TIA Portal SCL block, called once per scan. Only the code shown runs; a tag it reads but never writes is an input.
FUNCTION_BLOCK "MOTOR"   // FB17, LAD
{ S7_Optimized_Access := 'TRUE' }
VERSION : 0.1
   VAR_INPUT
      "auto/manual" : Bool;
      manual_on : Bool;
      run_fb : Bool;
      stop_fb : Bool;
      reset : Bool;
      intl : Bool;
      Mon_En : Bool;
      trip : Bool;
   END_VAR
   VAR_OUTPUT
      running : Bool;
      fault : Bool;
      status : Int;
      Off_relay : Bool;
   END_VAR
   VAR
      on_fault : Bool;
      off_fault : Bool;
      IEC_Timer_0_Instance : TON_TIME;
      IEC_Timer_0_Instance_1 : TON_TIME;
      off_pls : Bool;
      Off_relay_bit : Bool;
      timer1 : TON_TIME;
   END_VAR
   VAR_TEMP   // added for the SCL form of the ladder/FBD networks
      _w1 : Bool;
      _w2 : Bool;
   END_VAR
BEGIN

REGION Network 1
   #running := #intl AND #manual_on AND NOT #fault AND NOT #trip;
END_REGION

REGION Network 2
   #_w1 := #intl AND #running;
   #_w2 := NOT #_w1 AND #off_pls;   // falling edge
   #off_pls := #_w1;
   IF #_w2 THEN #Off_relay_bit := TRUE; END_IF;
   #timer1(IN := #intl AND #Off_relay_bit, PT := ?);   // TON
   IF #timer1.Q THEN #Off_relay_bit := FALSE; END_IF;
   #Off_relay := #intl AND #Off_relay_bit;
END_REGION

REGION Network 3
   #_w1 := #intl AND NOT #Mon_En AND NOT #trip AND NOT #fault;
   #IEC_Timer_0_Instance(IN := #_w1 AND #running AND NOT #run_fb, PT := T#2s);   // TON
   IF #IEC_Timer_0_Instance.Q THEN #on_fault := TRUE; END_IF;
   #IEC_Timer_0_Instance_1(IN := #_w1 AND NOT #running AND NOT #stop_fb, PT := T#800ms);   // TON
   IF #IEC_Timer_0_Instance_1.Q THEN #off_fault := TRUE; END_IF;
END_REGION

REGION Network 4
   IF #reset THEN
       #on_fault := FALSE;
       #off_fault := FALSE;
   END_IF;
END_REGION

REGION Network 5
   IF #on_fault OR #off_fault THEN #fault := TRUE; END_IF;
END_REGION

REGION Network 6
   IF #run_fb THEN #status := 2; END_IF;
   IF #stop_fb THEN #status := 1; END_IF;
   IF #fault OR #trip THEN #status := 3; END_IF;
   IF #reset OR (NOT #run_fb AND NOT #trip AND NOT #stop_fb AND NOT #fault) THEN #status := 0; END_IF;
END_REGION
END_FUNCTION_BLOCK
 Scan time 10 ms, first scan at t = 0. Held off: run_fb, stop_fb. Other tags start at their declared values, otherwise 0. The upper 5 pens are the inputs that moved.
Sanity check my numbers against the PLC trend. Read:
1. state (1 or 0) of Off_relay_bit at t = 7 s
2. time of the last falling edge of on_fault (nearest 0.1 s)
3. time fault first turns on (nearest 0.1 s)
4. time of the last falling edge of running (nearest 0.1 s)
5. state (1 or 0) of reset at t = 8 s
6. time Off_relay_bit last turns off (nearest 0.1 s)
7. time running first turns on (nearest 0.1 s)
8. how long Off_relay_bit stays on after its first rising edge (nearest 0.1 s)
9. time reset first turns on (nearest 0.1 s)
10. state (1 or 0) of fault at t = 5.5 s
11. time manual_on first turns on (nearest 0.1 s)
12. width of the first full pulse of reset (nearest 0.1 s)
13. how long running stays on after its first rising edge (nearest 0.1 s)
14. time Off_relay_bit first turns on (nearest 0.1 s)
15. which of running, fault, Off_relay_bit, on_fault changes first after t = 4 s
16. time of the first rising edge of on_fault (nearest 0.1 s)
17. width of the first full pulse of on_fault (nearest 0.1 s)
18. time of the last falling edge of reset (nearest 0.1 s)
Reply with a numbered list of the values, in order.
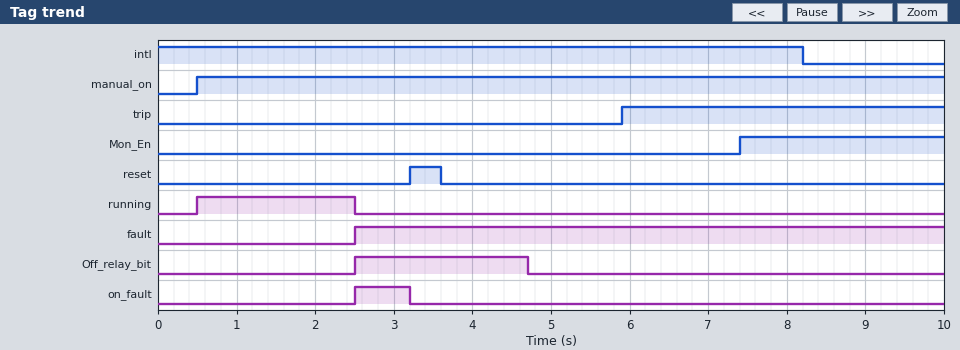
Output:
1. 0
2. 3.2 s
3. 2.5 s
4. 2.5 s
5. 0
6. 4.7 s
7. 0.5 s
8. 2.2 s
9. 3.2 s
10. 1
11. 0.5 s
12. 0.4 s
13. 2.0 s
14. 2.5 s
15. Off_relay_bit
16. 2.5 s
17. 0.7 s
18. 3.6 s
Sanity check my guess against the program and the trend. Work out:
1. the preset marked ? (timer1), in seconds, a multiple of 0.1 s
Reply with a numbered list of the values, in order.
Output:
1. 2.2 s
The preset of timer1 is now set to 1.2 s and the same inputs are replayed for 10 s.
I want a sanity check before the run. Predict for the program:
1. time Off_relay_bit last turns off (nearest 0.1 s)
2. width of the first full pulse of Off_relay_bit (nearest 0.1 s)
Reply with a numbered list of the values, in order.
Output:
1. 3.7 s
2. 1.2 s
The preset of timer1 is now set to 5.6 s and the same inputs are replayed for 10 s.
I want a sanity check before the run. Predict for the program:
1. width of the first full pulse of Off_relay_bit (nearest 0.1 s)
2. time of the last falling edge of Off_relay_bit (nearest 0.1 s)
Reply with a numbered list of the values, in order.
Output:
1. 5.6 s
2. 8.1 s
